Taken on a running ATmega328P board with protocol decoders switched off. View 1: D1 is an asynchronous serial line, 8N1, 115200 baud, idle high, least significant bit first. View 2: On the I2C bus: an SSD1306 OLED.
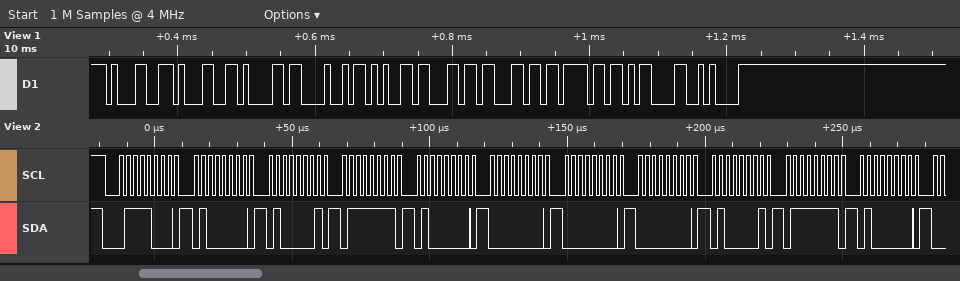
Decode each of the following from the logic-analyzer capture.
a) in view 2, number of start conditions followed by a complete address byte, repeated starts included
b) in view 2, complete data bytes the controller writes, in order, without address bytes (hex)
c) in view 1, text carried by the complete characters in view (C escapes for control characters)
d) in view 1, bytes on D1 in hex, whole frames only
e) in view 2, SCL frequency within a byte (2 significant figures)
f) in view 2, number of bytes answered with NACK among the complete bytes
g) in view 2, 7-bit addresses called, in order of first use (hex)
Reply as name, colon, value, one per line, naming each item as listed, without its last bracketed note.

in view 2, number of start conditions followed by a complete address byte, repeated starts included: 1
in view 2, complete data bytes the controller writes, in order, without address bytes: 40 41 7F 40 00 00 00 41 7F 40
in view 1, text carried by the complete characters in view: "11aHello\r\n"
in view 1, bytes on D1 in hex, whole frames only: 31 31 61 48 65 6C 6C 6F 0D 0A
in view 2, SCL frequency within a byte: 400 kHz
in view 2, number of bytes answered with NACK among the complete bytes: 0
in view 2, 7-bit addresses called, in order of first use: 0x3C
